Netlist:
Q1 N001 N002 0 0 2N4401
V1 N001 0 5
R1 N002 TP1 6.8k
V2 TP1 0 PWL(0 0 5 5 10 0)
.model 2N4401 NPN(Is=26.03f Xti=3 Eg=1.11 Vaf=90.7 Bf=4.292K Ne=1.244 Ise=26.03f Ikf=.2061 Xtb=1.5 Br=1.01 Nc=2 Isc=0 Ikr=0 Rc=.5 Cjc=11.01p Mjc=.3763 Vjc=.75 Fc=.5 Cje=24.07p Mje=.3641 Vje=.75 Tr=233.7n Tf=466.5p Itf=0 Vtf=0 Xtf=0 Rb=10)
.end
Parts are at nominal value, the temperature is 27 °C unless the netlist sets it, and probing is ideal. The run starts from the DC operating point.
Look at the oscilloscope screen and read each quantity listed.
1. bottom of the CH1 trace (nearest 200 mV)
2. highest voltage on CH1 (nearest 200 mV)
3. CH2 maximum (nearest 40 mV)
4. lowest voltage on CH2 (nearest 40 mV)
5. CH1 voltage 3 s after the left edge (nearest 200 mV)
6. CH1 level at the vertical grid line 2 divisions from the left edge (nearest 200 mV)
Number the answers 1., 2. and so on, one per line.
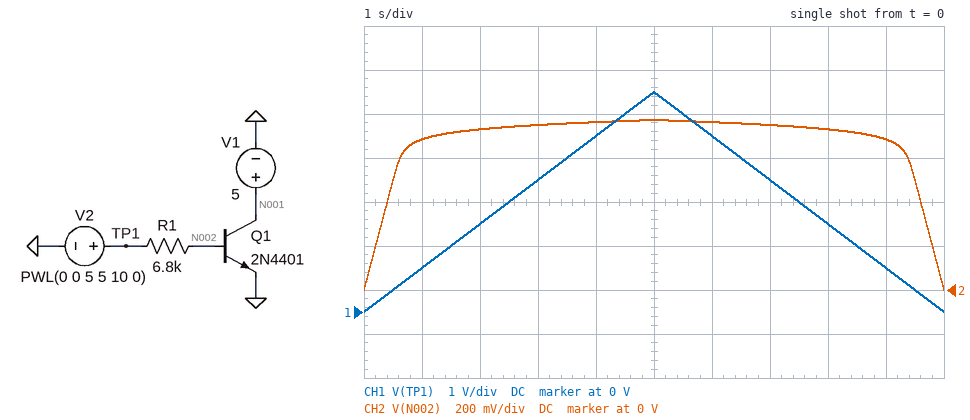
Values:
1. 0 V
2. 5.0 V
3. 760 mV
4. 0 V
5. 3.0 V
6. 2.0 V
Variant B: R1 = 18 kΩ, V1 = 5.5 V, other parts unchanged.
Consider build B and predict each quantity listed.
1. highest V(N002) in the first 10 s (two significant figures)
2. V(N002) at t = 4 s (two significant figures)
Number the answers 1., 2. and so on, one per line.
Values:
1. 740 mV
2. 730 mV
